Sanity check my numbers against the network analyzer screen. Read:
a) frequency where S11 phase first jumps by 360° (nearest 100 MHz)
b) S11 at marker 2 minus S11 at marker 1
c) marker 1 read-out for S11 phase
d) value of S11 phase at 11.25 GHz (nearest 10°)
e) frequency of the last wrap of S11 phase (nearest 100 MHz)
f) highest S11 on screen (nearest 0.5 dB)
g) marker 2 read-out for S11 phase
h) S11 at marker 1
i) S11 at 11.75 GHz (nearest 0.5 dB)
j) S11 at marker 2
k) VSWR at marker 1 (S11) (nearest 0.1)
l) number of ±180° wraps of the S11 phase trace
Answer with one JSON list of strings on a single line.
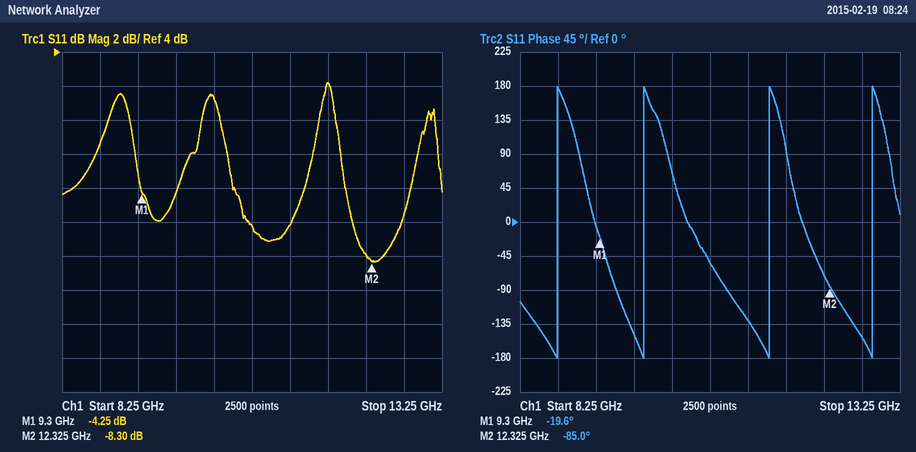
["8.7 GHz", "-4.05 dB", "-19.6°", "-130°", "12.9 GHz", "2.0 dB", "-85.0°", "-4.25 dB", "2.0 dB", "-8.30 dB", "4.2", "4"]
